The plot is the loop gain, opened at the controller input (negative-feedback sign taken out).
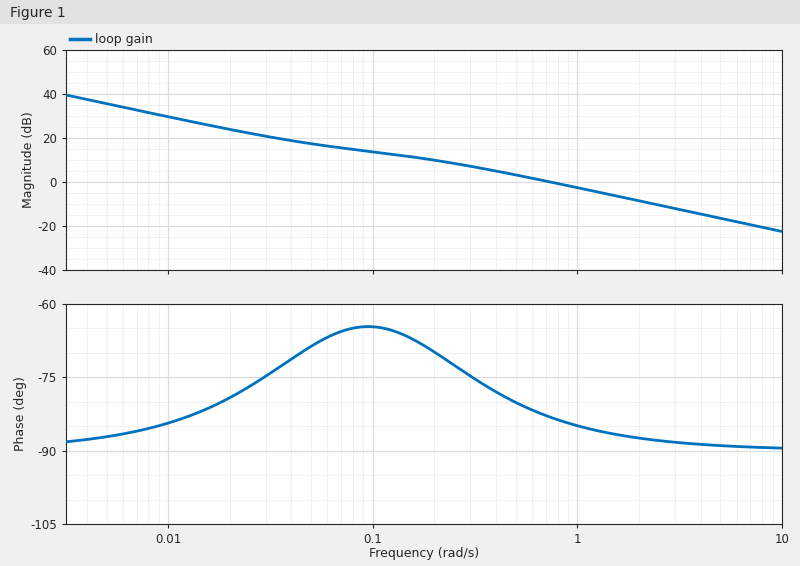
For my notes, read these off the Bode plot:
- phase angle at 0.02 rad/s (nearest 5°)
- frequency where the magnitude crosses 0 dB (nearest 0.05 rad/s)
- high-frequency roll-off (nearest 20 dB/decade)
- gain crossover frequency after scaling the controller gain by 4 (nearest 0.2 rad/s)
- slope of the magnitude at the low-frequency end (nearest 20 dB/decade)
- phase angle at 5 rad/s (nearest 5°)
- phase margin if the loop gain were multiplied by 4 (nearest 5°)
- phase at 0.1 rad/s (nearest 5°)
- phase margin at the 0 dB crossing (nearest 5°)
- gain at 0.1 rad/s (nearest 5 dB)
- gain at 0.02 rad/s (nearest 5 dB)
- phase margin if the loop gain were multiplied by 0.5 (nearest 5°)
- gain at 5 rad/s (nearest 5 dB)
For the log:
-80°
0.75 rad/s
-20 dB/decade
3.0 rad/s
-20 dB/decade
-90°
90°
-65°
95°
15 dB
25 dB
105°
-15 dB
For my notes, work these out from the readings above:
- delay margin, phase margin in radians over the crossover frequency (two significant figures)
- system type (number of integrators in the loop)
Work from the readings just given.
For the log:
2.2 s
1
